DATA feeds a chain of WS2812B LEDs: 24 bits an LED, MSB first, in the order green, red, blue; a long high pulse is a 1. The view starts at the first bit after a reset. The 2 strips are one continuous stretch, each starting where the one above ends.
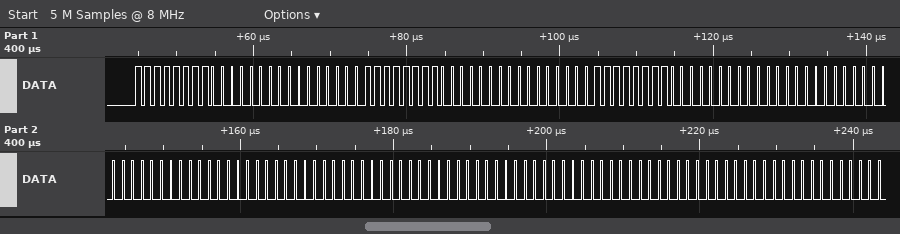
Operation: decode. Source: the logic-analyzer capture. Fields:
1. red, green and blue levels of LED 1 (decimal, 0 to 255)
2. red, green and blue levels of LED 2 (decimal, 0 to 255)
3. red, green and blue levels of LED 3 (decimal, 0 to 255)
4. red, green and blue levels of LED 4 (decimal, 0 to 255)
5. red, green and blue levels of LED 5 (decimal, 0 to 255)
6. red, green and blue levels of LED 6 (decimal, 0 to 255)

0, 255, 0
0, 255, 0
0, 255, 0
0, 0, 0
0, 0, 0
0, 0, 0
